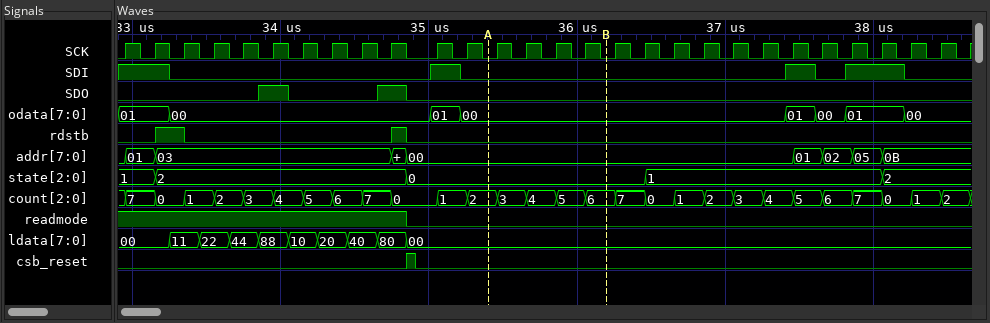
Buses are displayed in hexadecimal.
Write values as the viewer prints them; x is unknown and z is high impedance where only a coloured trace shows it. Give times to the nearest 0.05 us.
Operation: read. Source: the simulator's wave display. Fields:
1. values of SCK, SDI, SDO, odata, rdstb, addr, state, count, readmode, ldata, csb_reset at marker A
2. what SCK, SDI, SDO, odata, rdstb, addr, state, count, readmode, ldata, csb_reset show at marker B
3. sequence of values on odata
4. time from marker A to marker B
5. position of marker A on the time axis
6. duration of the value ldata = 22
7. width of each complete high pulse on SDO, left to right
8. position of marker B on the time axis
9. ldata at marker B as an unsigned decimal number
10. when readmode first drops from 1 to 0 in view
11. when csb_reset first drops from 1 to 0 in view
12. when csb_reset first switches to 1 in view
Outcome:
SCK=0, SDI=0, SDO=0, odata=00, rdstb=0, addr=00, state=0, count=2, readmode=0, ldata=00, csb_reset=0
SCK=0, SDI=0, SDO=0, odata=00, rdstb=0, addr=00, state=0, count=6, readmode=0, ldata=00, csb_reset=0
01, 00, 01, 00, 01, 00, 01, 00
0.8 us
35.4 us
0.2 us
0.2 us, 0.2 us
36.2 us
0
34.85 us
34.9 us
34.85 us
